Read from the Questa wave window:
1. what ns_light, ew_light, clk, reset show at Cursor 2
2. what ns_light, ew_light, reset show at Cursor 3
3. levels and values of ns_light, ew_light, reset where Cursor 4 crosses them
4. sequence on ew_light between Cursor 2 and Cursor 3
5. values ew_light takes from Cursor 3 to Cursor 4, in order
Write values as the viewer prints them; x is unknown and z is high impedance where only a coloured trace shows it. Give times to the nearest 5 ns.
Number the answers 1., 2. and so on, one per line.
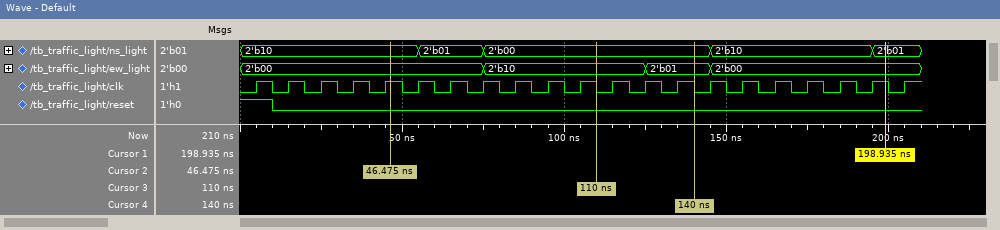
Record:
1. ns_light=2'b10, ew_light=2'b00, clk=1, reset=0
2. ns_light=2'b00, ew_light=2'b10, reset=0
3. ns_light=2'b00, ew_light=2'b01, reset=0
4. 2'b00, 2'b10
5. 2'b10, 2'b01
